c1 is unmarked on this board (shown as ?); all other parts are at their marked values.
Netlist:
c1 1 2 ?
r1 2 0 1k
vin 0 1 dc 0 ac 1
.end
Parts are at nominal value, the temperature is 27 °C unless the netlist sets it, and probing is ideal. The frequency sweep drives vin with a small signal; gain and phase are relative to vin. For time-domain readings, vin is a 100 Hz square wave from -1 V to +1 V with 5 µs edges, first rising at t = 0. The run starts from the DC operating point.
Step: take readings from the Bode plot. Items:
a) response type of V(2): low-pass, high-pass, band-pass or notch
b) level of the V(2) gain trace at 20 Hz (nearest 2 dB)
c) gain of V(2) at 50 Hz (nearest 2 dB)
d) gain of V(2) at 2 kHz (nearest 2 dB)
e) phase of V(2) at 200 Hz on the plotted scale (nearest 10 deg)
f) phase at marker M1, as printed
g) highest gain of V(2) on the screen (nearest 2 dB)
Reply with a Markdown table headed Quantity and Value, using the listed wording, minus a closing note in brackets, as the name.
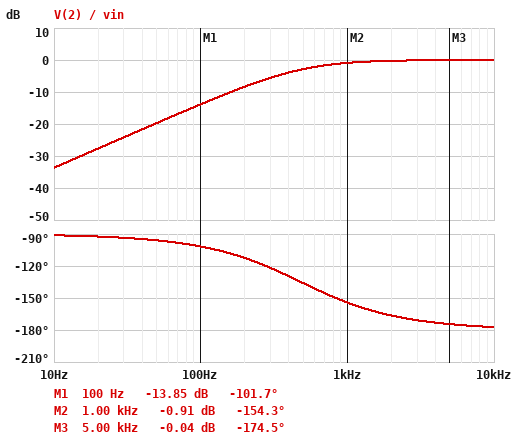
| Quantity | Value |
|---|---|
| response type of V(2): low-pass, high-pass, band-pass or notch | high-pass |
| level of the V(2) gain trace at 20 Hz | -28 dB |
| gain of V(2) at 50 Hz | -20 dB |
| gain of V(2) at 2 kHz | 0 dB |
| phase of V(2) at 200 Hz on the plotted scale | -110 deg |
| phase at marker M1, as printed | -101.7 deg |
| highest gain of V(2) on the screen | 0 dB |
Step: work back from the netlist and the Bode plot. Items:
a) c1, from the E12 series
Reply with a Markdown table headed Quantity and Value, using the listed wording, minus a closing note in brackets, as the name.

| Quantity | Value |
|---|---|
| c1, from the E12 series | 330 nF |
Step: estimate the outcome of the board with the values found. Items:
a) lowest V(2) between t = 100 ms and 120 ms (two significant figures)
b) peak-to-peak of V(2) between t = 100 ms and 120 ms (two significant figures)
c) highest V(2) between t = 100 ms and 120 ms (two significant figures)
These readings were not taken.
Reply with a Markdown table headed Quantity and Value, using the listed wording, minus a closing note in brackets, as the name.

| Quantity | Value |
|---|---|
| lowest V(2) between t = 100 ms and 120 ms | -2.0 V |
| peak-to-peak of V(2) between t = 100 ms and 120 ms | 4.0 V |
| highest V(2) between t = 100 ms and 120 ms | 2.0 V |
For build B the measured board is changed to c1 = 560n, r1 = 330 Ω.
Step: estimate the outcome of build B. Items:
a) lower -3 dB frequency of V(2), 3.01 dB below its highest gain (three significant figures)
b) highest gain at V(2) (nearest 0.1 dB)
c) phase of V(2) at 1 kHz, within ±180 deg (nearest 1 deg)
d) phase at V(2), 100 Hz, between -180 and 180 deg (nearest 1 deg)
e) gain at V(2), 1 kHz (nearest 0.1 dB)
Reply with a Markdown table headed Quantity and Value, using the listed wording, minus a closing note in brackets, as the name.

| Quantity | Value |
|---|---|
| lower -3 dB frequency of V(2), 3.01 dB below its highest gain | 861 Hz |
| highest gain at V(2) | 0 dB |
| phase of V(2) at 1 kHz, within ±180 deg | -139 deg |
| phase at V(2), 100 Hz, between -180 and 180 deg | -97 deg |
| gain at V(2), 1 kHz | -2.4 dB |
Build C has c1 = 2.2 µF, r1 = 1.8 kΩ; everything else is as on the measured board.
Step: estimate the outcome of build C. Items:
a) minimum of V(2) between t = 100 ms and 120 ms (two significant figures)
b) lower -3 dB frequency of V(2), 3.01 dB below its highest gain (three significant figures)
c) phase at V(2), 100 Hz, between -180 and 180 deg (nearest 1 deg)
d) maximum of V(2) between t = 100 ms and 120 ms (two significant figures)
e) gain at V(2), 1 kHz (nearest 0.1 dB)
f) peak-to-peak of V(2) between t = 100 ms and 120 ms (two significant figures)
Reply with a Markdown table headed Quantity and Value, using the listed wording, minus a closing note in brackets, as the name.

| Quantity | Value |
|---|---|
| minimum of V(2) between t = 100 ms and 120 ms | -1.6 V |
| lower -3 dB frequency of V(2), 3.01 dB below its highest gain | 40.2 Hz |
| phase at V(2), 100 Hz, between -180 and 180 deg | -158 deg |
| maximum of V(2) between t = 100 ms and 120 ms | 1.6 V |
| gain at V(2), 1 kHz | 0 dB |
| peak-to-peak of V(2) between t = 100 ms and 120 ms | 3.1 V |
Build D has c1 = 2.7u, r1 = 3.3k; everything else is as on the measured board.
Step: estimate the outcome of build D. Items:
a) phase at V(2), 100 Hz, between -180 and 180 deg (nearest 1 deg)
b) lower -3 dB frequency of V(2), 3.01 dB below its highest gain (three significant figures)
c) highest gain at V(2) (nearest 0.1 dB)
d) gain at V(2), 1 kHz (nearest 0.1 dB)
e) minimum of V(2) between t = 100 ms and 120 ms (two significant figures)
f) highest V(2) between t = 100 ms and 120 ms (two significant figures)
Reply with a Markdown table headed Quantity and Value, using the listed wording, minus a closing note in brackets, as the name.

| Quantity | Value |
|---|---|
| phase at V(2), 100 Hz, between -180 and 180 deg | -170 deg |
| lower -3 dB frequency of V(2), 3.01 dB below its highest gain | 17.9 Hz |
| highest gain at V(2) | 0 dB |
| gain at V(2), 1 kHz | 0 dB |
| minimum of V(2) between t = 100 ms and 120 ms | -1.3 V |
| highest V(2) between t = 100 ms and 120 ms | 1.3 V |
